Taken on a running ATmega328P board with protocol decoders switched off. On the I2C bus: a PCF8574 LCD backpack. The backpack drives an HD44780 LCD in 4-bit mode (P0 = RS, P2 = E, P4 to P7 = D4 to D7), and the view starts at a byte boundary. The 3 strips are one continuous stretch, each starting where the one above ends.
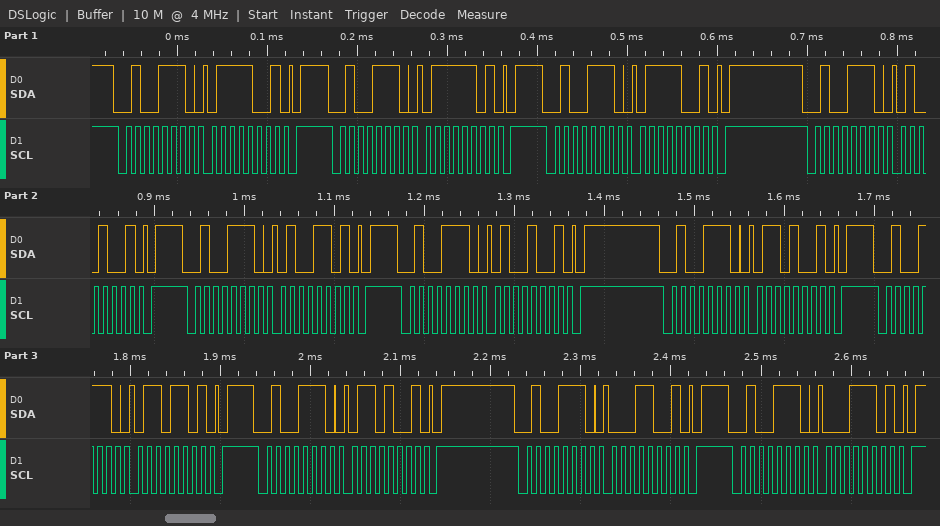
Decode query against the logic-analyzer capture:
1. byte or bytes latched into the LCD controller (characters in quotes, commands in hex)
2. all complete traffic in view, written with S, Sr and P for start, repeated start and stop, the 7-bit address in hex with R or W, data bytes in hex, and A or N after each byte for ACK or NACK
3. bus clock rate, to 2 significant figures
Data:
't'
S 27W A 79 A P S 27W A 7D A P S 27W A 79 A P S 27W A 49 A P S 27W A 4D A P S 27W A 49 A P S 27W A 69 A P S 27W A 6D A P S 27W A 69 A P S 27W A 19 A P S 27W A 1D A P
100 kHz
